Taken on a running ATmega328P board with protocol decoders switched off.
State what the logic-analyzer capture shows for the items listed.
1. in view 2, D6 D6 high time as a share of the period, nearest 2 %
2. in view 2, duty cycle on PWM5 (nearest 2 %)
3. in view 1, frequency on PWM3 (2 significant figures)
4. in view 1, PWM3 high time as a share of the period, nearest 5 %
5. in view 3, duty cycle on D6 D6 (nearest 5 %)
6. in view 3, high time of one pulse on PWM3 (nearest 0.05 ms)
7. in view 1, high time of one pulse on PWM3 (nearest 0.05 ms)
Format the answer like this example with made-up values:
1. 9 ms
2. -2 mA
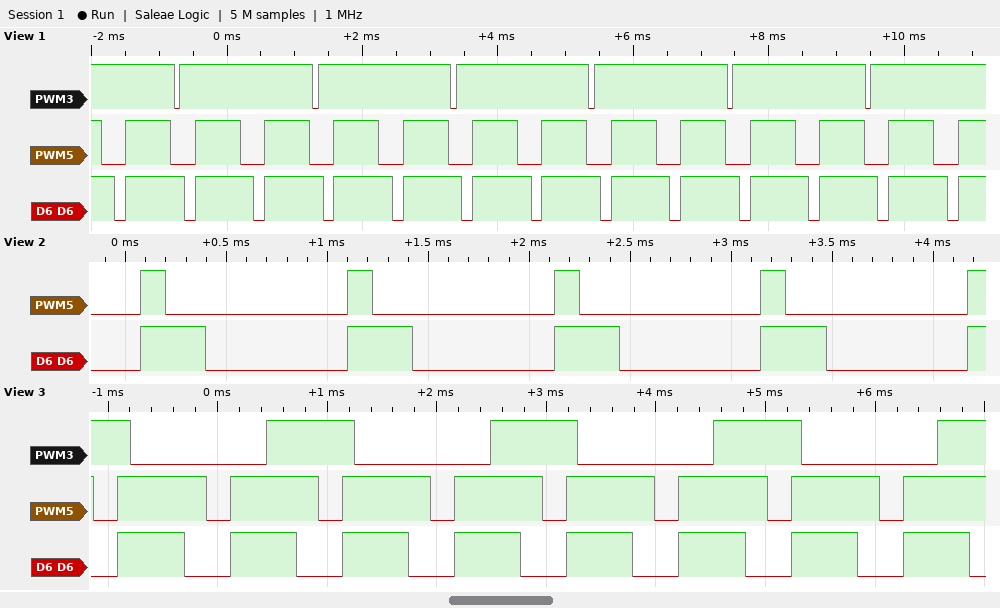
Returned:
1. 32 %
2. 12 %
3. 490 Hz
4. 95 %
5. 60 %
6. 0.80 ms
7. 1.95 ms
